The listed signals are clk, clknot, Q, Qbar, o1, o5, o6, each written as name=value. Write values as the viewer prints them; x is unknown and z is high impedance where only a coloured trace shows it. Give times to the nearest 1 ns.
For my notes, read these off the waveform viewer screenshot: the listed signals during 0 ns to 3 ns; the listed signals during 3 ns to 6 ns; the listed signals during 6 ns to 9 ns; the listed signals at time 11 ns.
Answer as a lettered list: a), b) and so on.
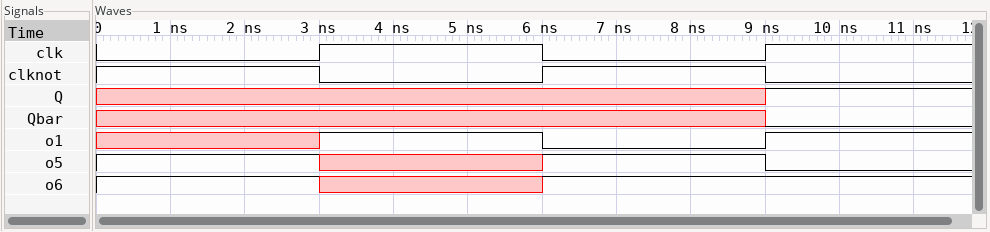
a) clk=0, clknot=1, Q=x, Qbar=x, o1=x, o5=1, o6=1
b) clk=1, clknot=0, Q=x, Qbar=x, o1=1, o5=x, o6=x
c) clk=0, clknot=1, Q=x, Qbar=x, o1=0, o5=1, o6=1
d) clk=1, clknot=0, Q=1, Qbar=0, o1=1, o5=0, o6=1
